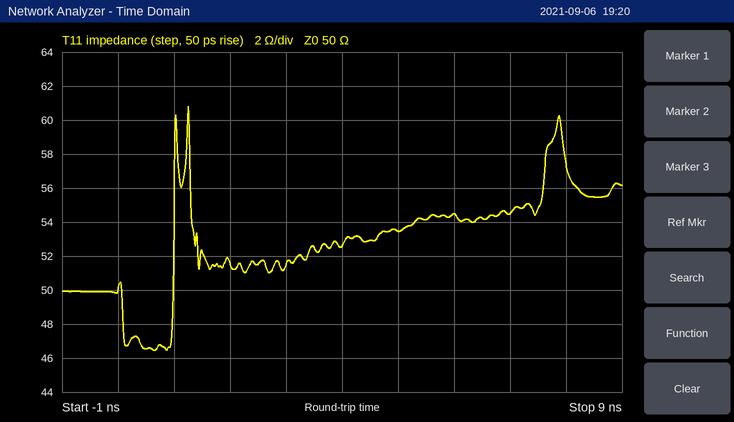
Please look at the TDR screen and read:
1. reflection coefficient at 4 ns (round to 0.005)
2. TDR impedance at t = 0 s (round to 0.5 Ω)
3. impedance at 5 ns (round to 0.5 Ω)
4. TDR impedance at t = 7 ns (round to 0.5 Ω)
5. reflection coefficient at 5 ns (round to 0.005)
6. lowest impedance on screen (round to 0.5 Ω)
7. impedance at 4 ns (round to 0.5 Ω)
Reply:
+0.025
50.0 Ω
53.5 Ω
54.5 Ω
+0.035
46.5 Ω
52.5 Ω
